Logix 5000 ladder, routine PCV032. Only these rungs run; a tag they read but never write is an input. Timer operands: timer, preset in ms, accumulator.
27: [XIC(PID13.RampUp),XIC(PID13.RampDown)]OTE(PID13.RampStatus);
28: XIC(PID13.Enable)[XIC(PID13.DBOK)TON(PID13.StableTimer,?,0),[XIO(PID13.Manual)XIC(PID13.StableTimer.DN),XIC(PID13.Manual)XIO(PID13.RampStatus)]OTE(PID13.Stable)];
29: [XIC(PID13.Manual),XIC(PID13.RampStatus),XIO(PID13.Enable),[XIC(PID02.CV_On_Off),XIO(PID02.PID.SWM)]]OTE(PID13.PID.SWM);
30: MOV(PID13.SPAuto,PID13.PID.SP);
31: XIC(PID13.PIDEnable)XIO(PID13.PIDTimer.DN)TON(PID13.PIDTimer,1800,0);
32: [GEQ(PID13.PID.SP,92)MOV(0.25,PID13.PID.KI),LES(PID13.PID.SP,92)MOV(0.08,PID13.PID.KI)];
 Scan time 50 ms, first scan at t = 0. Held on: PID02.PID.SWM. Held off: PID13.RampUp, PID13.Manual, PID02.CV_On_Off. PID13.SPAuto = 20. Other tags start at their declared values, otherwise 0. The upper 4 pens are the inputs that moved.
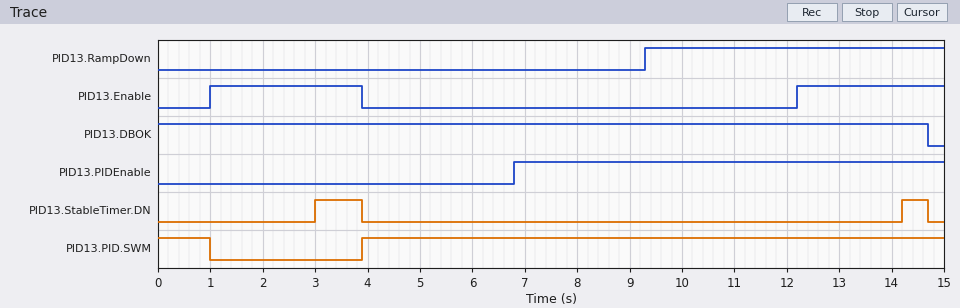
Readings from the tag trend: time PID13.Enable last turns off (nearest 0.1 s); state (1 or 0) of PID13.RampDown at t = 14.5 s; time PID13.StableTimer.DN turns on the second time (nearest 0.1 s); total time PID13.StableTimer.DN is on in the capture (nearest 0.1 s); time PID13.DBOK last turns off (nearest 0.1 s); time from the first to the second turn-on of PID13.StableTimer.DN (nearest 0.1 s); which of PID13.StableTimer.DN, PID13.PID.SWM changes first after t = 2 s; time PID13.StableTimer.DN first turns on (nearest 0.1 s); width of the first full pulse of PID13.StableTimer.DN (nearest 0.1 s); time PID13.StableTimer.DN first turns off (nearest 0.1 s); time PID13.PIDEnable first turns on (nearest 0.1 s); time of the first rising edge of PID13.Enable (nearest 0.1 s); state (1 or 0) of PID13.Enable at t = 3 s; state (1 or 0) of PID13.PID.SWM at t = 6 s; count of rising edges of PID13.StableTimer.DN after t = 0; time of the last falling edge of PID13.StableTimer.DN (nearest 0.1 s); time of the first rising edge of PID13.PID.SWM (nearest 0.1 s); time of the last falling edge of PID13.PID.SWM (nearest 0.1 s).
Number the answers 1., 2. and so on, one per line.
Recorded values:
1. 3.9 s
2. 1
3. 14.2 s
4. 1.4 s
5. 14.7 s
6. 11.2 s
7. PID13.StableTimer.DN
8. 3.0 s
9. 0.9 s
10. 3.9 s
11. 6.8 s
12. 1.0 s
13. 1
14. 1
15. 2
16. 14.7 s
17. 3.9 s
18. 1.0 s
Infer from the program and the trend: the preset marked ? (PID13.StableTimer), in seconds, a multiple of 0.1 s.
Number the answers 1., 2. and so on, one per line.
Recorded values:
1. 2.0 s
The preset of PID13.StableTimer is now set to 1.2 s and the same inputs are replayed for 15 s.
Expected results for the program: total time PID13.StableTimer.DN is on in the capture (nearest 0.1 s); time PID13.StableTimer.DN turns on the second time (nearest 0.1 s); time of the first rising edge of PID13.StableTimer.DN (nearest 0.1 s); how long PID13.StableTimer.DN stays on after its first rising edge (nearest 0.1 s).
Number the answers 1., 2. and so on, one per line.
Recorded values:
1. 3.0 s
2. 13.4 s
3. 2.2 s
4. 1.7 s
